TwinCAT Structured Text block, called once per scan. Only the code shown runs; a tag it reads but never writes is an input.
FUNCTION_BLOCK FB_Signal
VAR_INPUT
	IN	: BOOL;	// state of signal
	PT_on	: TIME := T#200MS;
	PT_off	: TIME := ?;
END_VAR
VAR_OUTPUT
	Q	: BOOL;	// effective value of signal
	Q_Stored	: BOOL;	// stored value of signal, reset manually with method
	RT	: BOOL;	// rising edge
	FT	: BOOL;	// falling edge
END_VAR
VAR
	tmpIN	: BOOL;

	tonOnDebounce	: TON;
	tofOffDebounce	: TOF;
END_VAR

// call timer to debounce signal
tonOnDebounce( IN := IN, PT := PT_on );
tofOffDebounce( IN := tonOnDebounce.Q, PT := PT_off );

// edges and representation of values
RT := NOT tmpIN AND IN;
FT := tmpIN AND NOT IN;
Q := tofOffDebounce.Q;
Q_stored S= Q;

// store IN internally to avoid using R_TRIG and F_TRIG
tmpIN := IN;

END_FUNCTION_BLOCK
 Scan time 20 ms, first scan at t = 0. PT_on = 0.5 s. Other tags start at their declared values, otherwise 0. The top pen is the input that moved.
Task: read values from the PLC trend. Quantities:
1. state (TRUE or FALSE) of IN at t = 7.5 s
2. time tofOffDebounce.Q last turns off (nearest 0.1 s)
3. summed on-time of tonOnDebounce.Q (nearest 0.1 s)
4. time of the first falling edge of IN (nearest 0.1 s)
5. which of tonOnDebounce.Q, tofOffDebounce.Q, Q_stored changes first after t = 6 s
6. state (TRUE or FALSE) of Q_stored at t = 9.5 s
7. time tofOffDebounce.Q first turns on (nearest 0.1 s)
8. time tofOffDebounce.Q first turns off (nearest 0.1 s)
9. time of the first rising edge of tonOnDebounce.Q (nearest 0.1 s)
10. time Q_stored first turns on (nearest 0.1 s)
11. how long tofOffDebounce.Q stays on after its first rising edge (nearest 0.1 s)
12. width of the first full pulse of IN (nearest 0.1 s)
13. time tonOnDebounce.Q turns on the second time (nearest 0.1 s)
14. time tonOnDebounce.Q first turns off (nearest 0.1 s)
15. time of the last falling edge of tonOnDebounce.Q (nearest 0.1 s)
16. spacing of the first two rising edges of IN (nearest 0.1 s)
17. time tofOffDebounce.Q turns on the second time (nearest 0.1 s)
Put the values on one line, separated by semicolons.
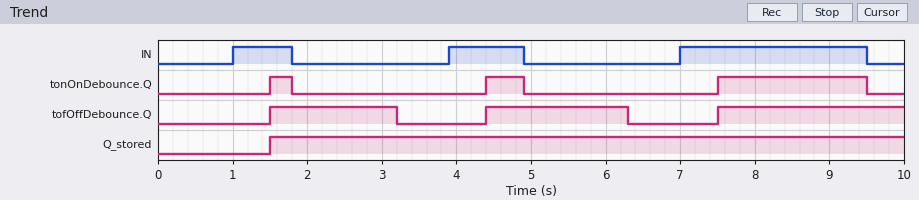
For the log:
TRUE; 6.3 s; 2.8 s; 1.8 s; tofOffDebounce.Q; TRUE; 1.5 s; 3.2 s; 1.5 s; 1.5 s; 1.7 s; 0.8 s; 4.4 s; 1.8 s; 9.5 s; 2.9 s; 4.4 s
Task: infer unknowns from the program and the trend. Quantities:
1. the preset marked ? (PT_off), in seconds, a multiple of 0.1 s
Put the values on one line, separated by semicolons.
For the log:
1.4 s
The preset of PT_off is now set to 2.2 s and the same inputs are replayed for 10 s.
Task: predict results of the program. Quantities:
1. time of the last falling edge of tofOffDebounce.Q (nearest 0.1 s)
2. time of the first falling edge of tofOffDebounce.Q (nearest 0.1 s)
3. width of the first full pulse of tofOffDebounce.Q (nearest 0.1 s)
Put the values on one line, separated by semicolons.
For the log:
7.1 s; 4.0 s; 2.5 s
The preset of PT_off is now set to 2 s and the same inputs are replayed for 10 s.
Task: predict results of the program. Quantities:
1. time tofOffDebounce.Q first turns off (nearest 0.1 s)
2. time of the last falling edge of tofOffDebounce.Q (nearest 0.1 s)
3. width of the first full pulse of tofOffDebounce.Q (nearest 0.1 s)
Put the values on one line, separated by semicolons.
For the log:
3.8 s; 6.9 s; 2.3 s
